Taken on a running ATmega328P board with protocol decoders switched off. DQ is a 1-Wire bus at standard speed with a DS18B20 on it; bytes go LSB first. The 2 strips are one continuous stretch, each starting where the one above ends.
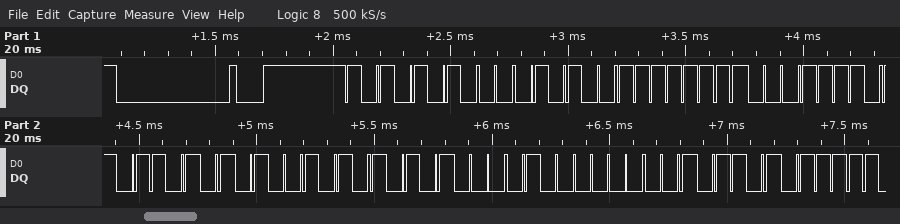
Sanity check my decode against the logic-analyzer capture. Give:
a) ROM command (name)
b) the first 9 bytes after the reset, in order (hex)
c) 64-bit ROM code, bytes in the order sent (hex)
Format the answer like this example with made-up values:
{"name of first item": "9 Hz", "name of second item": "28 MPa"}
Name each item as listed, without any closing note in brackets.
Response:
{"ROM command": "Match ROM", "the first 9 bytes after the reset, in order": "55 28 FF 78 AD 52 15 02 B4", "64-bit ROM code, bytes in the order sent": "28 FF 78 AD 52 15 02 B4"}
